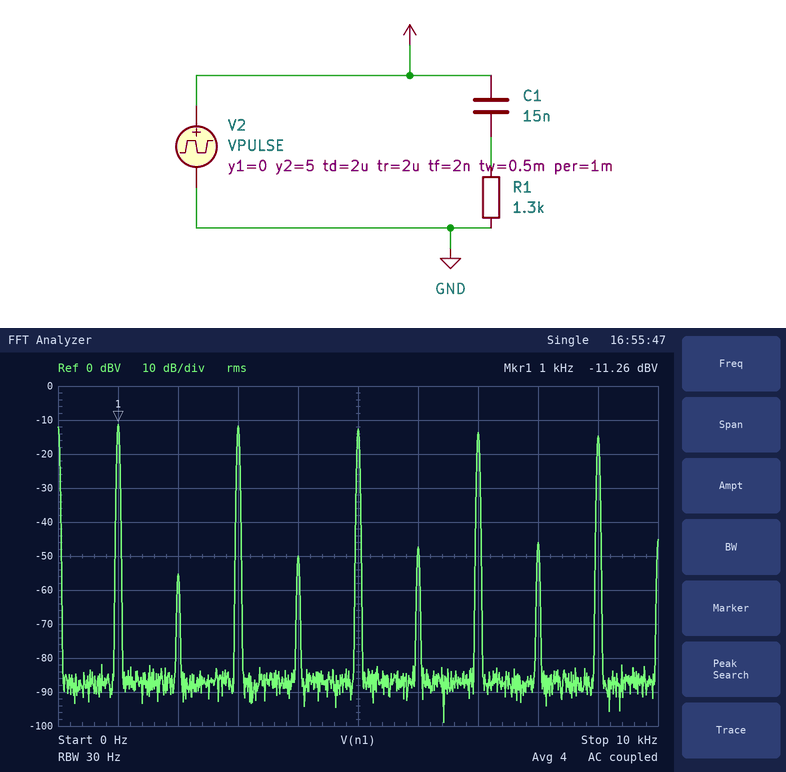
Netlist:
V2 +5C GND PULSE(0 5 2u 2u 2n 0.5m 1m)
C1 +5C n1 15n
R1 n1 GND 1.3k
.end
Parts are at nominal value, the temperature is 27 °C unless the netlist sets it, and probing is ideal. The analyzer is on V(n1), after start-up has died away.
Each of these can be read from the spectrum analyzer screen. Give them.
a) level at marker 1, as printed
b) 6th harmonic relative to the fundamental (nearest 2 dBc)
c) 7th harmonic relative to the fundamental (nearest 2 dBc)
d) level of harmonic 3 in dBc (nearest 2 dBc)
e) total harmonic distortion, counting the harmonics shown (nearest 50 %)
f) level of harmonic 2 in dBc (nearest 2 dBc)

-11.26 dBV
-36 dBc
-2 dBc
0 dBc
150 %
-44 dBc
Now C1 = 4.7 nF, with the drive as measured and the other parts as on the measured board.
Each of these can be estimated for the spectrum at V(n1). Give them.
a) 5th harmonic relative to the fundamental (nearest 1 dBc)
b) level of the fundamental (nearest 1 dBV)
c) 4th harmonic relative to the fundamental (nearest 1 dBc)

0 dBc
-21 dBV
-38 dBc
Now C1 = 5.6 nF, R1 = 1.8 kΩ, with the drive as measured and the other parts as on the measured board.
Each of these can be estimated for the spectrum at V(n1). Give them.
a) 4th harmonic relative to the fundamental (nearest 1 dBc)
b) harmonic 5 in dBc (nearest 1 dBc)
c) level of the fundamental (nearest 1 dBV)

-38 dBc
0 dBc
-17 dBV
